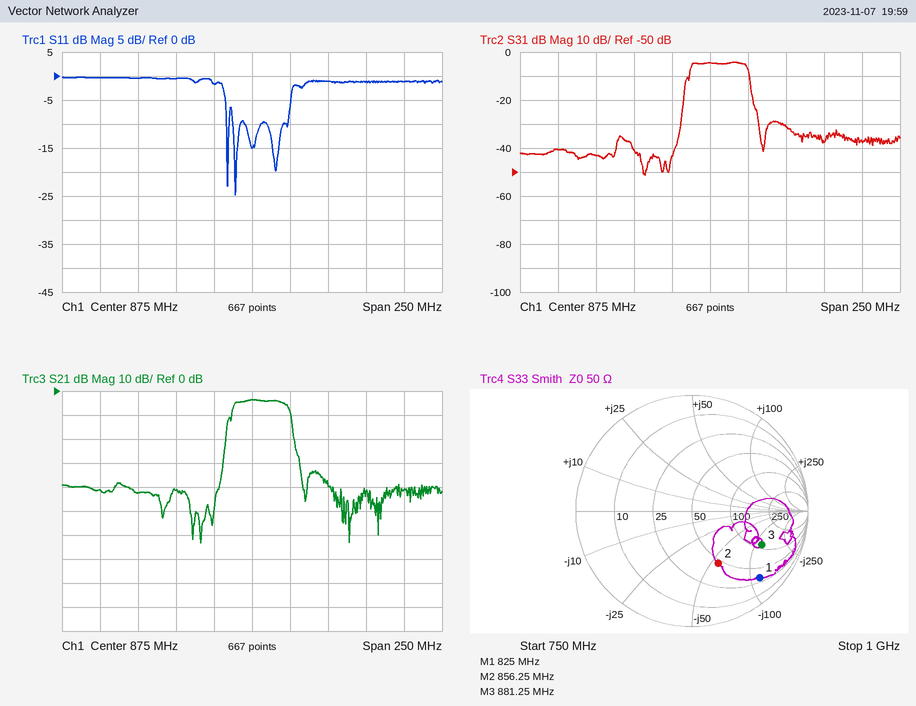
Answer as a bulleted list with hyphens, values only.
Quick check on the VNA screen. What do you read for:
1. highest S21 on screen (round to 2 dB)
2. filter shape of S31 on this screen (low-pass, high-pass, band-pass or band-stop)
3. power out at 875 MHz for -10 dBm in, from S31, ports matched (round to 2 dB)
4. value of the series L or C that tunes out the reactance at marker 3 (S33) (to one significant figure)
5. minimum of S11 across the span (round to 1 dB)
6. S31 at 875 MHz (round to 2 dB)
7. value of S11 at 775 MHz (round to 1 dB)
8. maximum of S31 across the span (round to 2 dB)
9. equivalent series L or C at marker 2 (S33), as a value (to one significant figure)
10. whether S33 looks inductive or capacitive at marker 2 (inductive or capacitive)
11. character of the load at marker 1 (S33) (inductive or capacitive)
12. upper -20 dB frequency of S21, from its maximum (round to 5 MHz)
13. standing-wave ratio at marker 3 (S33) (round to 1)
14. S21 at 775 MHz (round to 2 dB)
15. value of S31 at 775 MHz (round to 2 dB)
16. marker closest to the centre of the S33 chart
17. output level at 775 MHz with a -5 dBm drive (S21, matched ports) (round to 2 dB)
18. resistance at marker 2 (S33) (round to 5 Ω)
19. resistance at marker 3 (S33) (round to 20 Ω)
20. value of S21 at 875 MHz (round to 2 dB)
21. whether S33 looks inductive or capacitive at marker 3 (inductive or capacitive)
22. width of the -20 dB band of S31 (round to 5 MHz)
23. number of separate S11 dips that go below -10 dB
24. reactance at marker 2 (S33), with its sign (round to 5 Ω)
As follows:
- -4 dB
- band-pass
- -14 dBm
- 20 nH
- -25 dB
- -4 dB
- 0 dB
- -4 dB
- 3 pF
- capacitive
- capacitive
- 905 MHz
- 5
- -42 dB
- -40 dB
- marker 2
- -46 dBm
- 45 Ω
- 120 Ω
- -4 dB
- capacitive
- 50 MHz
- 4
- -55 Ω
